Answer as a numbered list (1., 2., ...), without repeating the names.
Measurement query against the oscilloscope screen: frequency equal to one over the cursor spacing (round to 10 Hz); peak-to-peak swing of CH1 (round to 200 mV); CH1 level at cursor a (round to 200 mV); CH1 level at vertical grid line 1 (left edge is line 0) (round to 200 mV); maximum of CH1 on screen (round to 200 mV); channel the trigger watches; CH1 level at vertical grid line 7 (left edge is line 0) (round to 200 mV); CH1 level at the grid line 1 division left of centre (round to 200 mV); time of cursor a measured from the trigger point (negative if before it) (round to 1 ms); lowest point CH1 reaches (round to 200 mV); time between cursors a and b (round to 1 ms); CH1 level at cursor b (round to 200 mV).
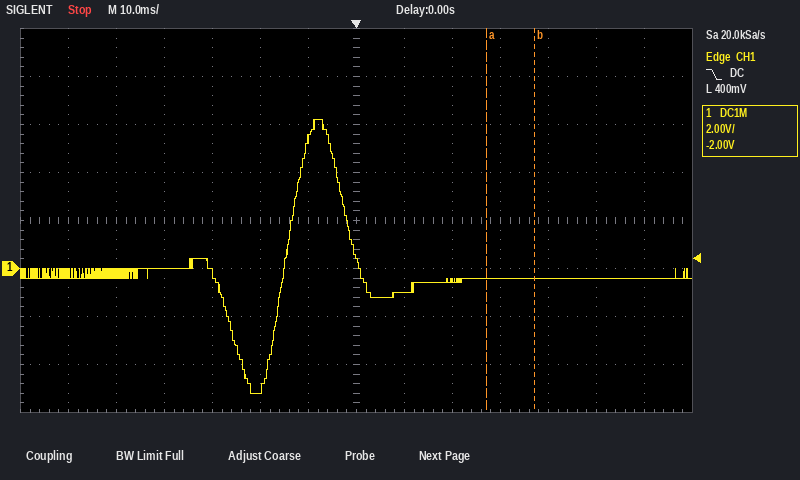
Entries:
1. 100 Hz
2. 11.4 V
3. -400 mV
4. -200 mV
5. 6.2 V
6. CH1
7. 400 mV
8. 5.4 V
9. +27 ms
10. -5.2 V
11. 10 ms
12. -400 mV
